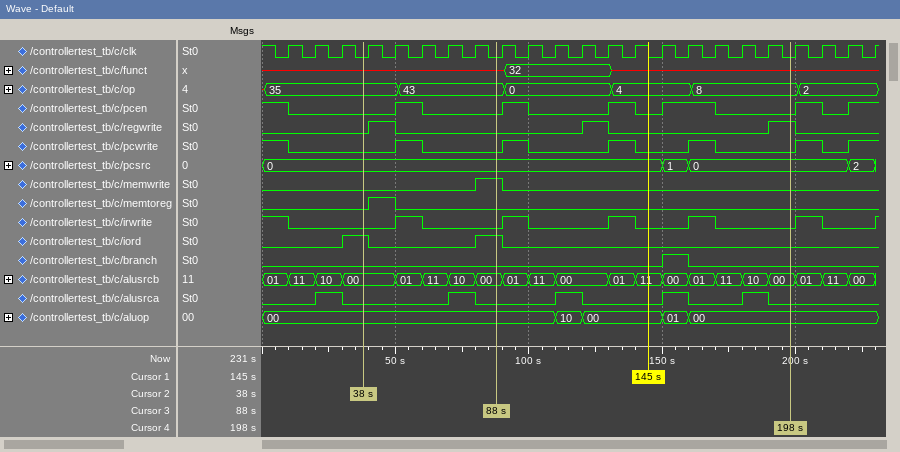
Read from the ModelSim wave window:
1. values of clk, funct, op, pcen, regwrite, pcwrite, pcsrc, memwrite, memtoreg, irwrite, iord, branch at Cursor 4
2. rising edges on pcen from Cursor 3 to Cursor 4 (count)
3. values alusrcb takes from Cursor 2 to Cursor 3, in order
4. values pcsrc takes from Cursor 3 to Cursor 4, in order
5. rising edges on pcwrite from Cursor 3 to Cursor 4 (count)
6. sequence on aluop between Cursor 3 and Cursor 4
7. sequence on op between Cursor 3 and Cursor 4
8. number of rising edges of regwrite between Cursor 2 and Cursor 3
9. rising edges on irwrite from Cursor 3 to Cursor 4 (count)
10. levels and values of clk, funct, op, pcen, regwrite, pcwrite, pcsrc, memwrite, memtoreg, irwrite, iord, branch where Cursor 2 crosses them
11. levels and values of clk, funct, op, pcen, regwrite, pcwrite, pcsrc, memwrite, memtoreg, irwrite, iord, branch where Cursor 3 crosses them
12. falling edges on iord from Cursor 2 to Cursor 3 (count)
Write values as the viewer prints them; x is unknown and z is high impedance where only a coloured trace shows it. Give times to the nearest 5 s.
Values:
clk=0, funct=x, op=8, pcen=0, regwrite=1, pcwrite=0, pcsrc=0, memwrite=0, memtoreg=0, irwrite=0, iord=0, branch=0
3
00, 01, 11, 10, 00
0, 1, 0
3
00, 10, 00, 01, 00
43, 0, 4, 8
1
3
clk=0, funct=x, op=35, pcen=0, regwrite=0, pcwrite=0, pcsrc=0, memwrite=0, memtoreg=0, irwrite=0, iord=1, branch=0
clk=0, funct=x, op=43, pcen=0, regwrite=0, pcwrite=0, pcsrc=0, memwrite=1, memtoreg=0, irwrite=0, iord=1, branch=0
1
